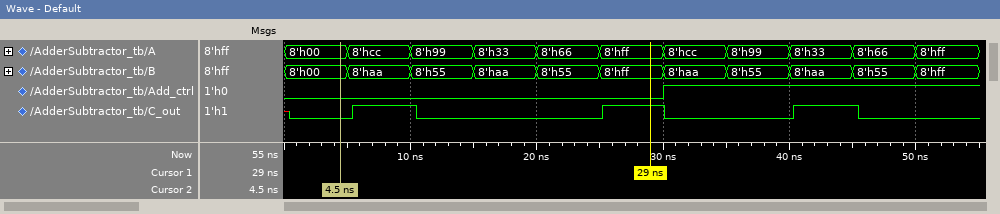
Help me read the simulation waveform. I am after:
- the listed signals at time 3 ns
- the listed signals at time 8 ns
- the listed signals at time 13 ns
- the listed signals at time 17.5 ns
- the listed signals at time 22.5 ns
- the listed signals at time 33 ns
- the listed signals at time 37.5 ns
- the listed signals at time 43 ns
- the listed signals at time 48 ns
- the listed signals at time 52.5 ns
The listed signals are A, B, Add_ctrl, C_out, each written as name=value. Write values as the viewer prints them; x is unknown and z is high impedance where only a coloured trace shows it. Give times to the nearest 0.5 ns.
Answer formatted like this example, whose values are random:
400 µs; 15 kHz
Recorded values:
A=8'h00, B=8'h00, Add_ctrl=0, C_out=0; A=8'hcc, B=8'haa, Add_ctrl=0, C_out=1; A=8'h99, B=8'h55, Add_ctrl=0, C_out=0; A=8'h33, B=8'haa, Add_ctrl=0, C_out=0; A=8'h66, B=8'h55, Add_ctrl=0, C_out=0; A=8'hcc, B=8'haa, Add_ctrl=1, C_out=0; A=8'h99, B=8'h55, Add_ctrl=1, C_out=0; A=8'h33, B=8'haa, Add_ctrl=1, C_out=1; A=8'h66, B=8'h55, Add_ctrl=1, C_out=0; A=8'hff, B=8'hff, Add_ctrl=1, C_out=0
